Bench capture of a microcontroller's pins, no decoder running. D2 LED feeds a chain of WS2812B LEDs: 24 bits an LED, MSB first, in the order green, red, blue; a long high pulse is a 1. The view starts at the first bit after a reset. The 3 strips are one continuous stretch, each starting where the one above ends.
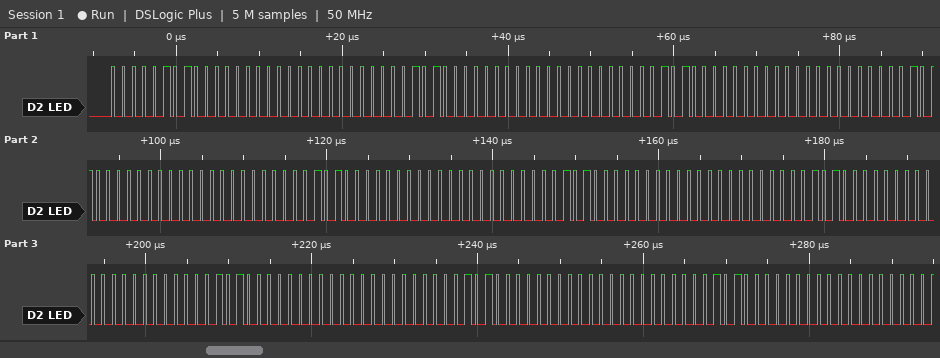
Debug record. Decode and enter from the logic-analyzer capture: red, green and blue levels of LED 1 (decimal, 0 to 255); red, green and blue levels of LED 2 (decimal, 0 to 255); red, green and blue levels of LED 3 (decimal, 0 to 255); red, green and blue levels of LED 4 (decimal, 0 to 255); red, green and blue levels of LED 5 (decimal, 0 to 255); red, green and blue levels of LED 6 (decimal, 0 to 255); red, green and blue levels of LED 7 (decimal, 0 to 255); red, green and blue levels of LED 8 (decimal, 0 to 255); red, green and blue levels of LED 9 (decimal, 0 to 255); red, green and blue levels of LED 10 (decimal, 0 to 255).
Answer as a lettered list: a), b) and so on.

a) 0, 5, 0
b) 0, 5, 0
c) 0, 5, 0
d) 0, 5, 0
e) 0, 5, 0
f) 0, 5, 0
g) 0, 5, 0
h) 0, 5, 0
i) 0, 5, 0
j) 0, 5, 0
